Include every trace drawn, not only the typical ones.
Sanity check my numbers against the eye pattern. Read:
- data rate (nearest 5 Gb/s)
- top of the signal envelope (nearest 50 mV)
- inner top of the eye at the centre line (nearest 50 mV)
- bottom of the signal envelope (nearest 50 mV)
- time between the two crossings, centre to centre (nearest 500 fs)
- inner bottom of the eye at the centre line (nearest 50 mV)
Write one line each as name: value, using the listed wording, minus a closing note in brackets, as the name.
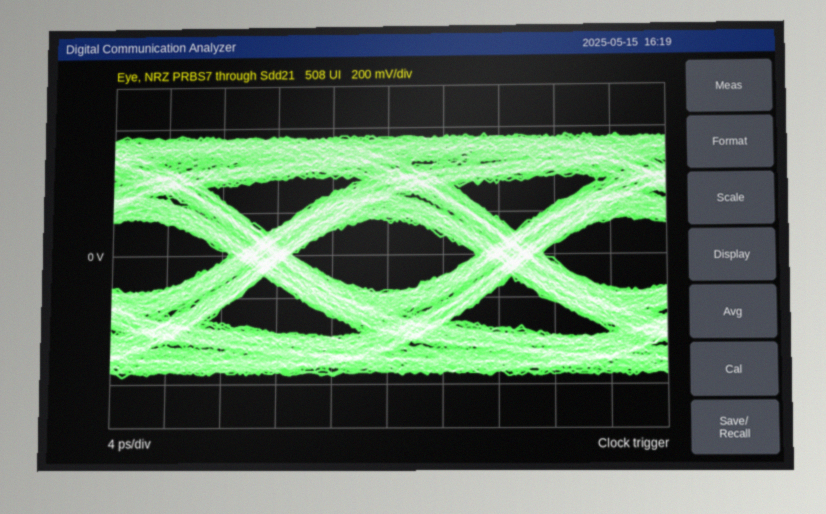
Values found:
data rate: 55 Gb/s
top of the signal envelope: 550 mV
inner top of the eye at the centre line: 150 mV
bottom of the signal envelope: -550 mV
time between the two crossings, centre to centre: 18.0 ps
inner bottom of the eye at the centre line: -150 mV
